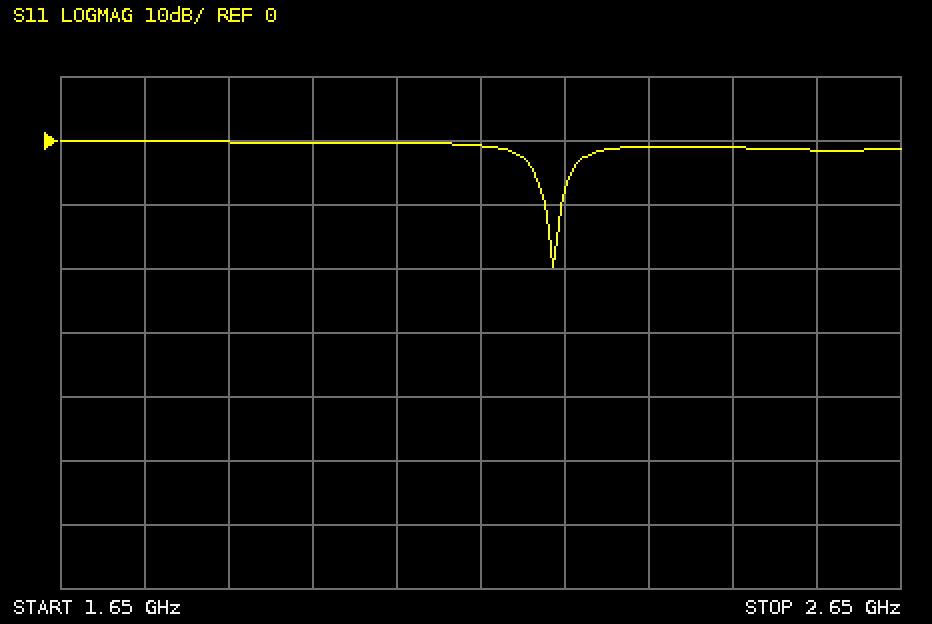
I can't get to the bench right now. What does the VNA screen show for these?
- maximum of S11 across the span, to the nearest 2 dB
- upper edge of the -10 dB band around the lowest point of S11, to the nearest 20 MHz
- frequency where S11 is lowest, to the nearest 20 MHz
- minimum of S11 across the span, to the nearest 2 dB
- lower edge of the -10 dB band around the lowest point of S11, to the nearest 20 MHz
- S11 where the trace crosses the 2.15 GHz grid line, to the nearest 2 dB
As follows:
0 dB
2.24 GHz
2.24 GHz
-20 dB
2.22 GHz
0 dB
